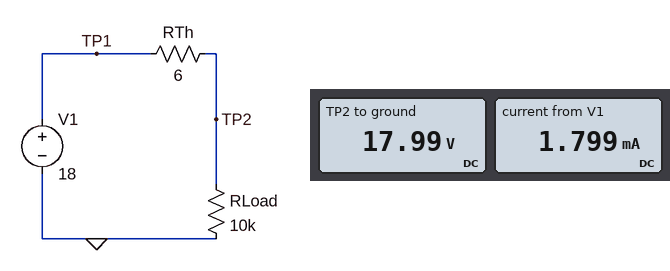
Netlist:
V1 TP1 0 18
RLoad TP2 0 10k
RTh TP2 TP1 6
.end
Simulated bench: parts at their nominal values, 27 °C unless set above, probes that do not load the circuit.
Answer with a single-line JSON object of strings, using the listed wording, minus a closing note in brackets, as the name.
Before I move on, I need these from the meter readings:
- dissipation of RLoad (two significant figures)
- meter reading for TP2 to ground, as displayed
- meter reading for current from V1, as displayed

{"dissipation of RLoad": "32 mW", "meter reading for TP2 to ground, as displayed": "17.99 V", "meter reading for current from V1, as displayed": "1.799 mA"}
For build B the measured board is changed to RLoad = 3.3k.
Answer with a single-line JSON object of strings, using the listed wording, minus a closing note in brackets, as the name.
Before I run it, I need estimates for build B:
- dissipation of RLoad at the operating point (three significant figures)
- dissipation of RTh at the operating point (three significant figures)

{"dissipation of RLoad at the operating point": "97.8 mW", "dissipation of RTh at the operating point": "178 µW"}
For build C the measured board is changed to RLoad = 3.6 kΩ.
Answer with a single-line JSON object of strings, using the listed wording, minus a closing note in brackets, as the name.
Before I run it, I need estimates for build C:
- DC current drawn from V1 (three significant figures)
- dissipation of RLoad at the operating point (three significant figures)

{"DC current drawn from V1": "4.99 mA", "dissipation of RLoad at the operating point": "89.7 mW"}
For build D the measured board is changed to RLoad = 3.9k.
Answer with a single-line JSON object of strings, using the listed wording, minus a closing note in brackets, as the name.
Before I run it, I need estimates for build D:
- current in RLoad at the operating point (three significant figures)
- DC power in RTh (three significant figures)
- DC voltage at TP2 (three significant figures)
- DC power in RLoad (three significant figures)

{"current in RLoad at the operating point": "4.61 mA", "DC power in RTh": "127 µW", "DC voltage at TP2": "18.0 V", "DC power in RLoad": "82.8 mW"}
